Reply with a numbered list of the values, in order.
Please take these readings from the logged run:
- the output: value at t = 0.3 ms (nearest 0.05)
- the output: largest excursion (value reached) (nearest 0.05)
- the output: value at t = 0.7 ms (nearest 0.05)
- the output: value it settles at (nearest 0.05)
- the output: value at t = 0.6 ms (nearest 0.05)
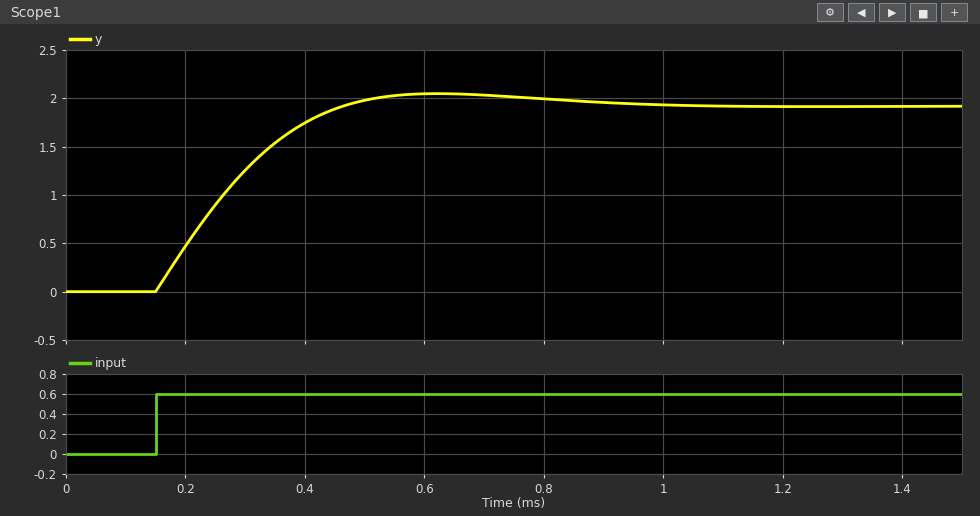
1. 1.25
2. 2.05
3. 2.05
4. 1.90
5. 2.05
